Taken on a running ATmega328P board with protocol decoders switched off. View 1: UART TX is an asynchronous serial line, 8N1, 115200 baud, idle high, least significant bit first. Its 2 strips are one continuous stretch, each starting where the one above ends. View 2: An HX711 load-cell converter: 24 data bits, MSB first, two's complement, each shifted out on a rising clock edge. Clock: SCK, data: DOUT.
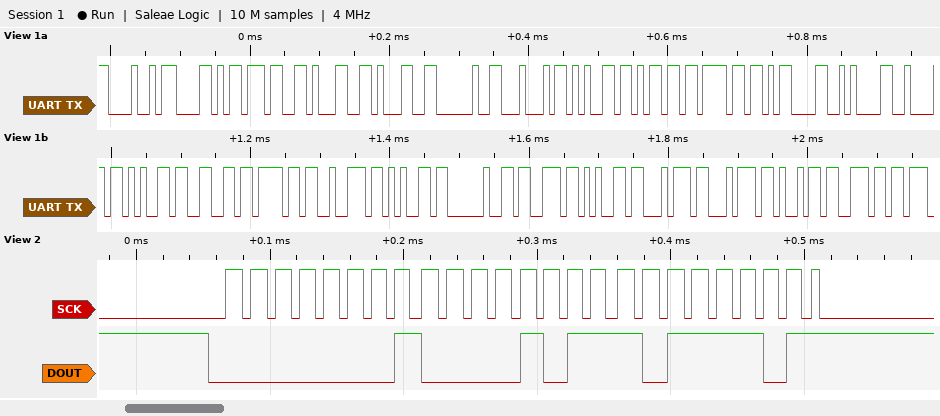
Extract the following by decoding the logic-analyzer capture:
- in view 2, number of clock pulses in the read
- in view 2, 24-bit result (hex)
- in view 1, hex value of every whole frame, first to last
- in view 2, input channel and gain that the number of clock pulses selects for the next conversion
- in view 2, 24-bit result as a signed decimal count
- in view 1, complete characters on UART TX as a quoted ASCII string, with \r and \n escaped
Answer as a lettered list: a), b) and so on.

a) 25
b) 0x010BBD
c) 0x48 0x58 0x37 0x31 0x31 0x20 0x44 0x65 0x6D 0x6F 0x0D 0x0A 0x42 0x65 0x66 0x6F 0x72 0x65 0x20 0x73 0x65 0x74 0x74 0x69 0x6E
d) channel A, gain 128
e) 68541
f) "HX711 Demo\r\nBefore settin"
